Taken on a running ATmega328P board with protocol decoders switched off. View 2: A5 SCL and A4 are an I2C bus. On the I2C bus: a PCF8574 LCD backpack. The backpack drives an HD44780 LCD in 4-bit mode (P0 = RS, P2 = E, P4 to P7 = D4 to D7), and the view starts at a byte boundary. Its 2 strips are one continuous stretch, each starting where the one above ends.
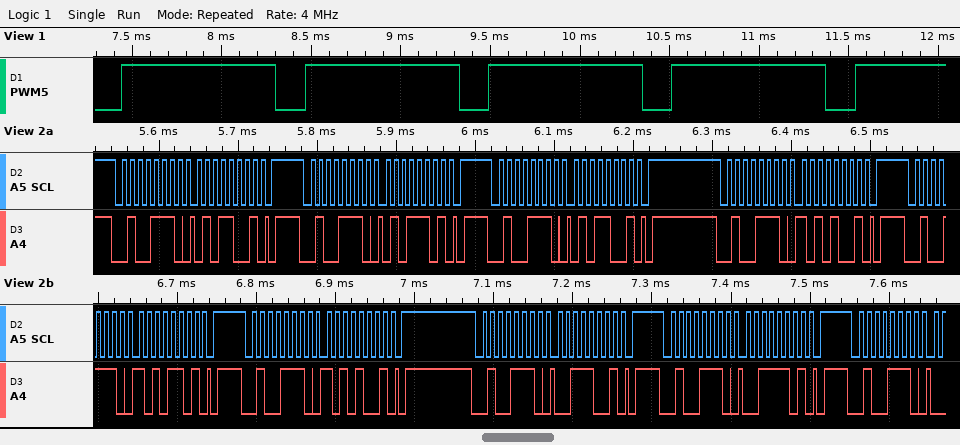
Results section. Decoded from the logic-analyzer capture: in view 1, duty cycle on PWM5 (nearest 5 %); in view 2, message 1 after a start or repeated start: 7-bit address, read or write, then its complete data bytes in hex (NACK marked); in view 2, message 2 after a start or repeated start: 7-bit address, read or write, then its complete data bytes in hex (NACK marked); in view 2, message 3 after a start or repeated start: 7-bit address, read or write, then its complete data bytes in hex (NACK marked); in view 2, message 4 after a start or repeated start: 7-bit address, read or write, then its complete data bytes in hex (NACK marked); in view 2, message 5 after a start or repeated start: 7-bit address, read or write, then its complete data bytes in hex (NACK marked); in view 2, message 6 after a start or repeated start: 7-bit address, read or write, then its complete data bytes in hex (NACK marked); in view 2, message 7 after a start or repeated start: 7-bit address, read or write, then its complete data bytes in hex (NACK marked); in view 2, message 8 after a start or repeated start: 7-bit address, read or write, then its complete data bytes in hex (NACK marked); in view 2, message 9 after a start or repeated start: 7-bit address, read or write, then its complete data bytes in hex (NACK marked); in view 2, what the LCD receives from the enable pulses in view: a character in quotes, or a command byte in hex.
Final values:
85 %
0x27 write: 59
0x27 write: 5D
0x27 write: 59
0x27 write: A9
0x27 write: AD
0x27 write: A9
0x27 write: 39
0x27 write: 3D
0x27 write
'Z'
